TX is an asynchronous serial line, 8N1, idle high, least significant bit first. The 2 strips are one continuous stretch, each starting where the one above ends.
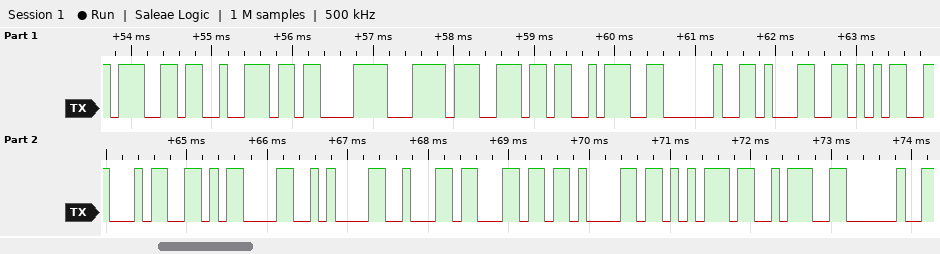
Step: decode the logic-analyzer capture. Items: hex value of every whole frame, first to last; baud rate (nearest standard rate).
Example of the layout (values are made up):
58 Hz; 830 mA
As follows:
0x67 0x72 0xC3 0xBC 0x6E 0x3A 0x20 0x31 0x35 0x34 0x0D 0x0A 0x62 0x6C 0x61 0x75 0x3A 0x20; 9600 baud
